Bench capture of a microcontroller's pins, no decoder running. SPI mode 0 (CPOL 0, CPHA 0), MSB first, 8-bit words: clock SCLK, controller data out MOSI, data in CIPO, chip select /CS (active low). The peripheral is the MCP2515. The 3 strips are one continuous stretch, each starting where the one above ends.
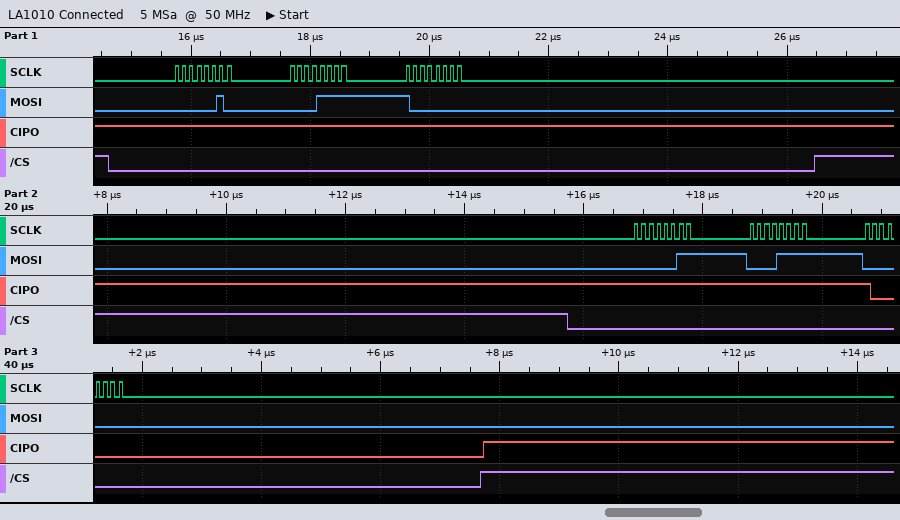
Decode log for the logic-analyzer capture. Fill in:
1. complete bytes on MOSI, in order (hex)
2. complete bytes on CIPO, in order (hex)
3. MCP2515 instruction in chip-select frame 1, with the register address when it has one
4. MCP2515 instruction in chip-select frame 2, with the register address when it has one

02 0F 80 03 0F 00
FF FF FF FF FF 80
WRITE 0x0F
READ 0x0F
